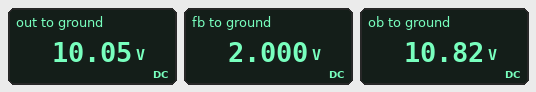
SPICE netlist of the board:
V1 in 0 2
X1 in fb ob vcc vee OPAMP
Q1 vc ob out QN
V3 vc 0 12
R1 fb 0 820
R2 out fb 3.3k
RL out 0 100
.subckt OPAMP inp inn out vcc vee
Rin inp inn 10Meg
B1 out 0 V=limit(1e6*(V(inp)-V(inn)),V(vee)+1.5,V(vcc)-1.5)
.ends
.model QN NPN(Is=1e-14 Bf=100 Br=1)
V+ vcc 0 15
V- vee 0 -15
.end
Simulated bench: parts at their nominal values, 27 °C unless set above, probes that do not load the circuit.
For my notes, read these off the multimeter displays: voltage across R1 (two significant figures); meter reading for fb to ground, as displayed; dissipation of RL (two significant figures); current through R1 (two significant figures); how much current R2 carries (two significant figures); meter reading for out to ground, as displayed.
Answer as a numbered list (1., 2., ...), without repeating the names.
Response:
1. 2.0 V
2. 2.000 V
3. 1.0 W
4. 2.4 mA
5. 2.4 mA
6. 10.05 V
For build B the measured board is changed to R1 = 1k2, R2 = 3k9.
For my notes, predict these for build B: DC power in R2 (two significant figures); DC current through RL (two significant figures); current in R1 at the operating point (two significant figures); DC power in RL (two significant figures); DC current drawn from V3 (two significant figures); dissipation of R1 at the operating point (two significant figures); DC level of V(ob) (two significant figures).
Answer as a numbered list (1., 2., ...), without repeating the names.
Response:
1. 11 mW
2. 85 mA
3. 1.7 mA
4. 720 mW
5. 86 mA
6. 3.3 mW
7. 9.3 V
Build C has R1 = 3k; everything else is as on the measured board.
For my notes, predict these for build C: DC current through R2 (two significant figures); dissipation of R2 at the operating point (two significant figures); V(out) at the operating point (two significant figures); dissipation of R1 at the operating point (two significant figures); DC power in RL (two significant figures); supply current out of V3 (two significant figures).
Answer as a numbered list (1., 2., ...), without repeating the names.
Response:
1. 670 µA
2. 1.5 mW
3. 4.2 V
4. 1.3 mW
5. 180 mW
6. 42 mA
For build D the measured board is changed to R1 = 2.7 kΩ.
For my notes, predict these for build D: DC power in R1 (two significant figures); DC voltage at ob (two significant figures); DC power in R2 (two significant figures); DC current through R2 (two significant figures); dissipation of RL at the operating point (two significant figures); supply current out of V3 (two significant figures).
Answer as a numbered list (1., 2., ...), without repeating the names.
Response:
1. 1.5 mW
2. 5.2 V
3. 1.8 mW
4. 740 µA
5. 200 mW
6. 45 mA
